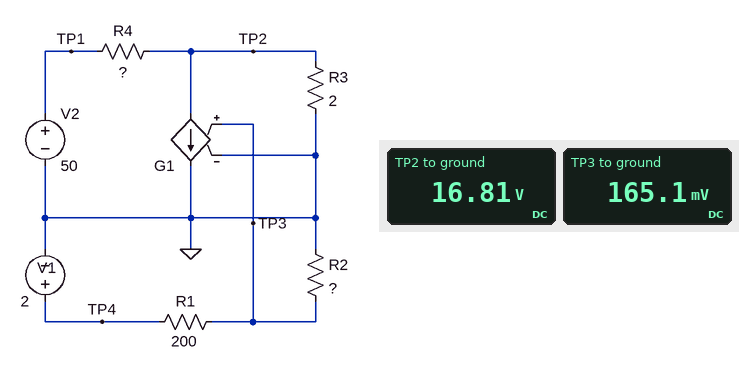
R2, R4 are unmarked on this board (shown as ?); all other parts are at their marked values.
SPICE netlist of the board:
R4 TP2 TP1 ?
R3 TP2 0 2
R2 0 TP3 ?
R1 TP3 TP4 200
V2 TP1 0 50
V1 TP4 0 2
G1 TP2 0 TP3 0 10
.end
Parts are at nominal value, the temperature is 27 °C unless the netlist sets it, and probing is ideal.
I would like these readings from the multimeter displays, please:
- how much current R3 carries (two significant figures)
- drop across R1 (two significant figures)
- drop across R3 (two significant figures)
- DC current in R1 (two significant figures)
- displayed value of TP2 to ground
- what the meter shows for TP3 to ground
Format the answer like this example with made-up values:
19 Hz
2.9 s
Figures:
8.4 A
1.8 V
17 V
9.2 mA
16.81 V
165.1 mV
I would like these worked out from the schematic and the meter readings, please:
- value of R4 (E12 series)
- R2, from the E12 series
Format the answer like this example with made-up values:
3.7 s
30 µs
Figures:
3.3 Ω
18 Ω
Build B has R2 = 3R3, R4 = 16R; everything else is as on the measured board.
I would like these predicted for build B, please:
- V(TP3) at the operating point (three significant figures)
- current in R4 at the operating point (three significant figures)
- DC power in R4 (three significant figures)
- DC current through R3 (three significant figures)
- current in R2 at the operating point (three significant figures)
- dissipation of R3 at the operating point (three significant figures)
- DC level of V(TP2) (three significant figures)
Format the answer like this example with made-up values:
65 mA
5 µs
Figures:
32.5 mV
2.81 A
127 W
2.49 A
9.84 mA
12.4 W
4.98 V
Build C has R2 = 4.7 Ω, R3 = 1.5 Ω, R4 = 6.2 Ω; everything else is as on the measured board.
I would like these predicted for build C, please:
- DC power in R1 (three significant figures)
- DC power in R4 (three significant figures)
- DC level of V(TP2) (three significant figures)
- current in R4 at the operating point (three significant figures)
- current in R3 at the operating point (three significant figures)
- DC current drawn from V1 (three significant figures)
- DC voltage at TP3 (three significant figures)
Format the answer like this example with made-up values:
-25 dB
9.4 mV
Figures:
19.1 mW
269 W
9.19 V
6.58 A
6.12 A
9.77 mA
45.9 mV
